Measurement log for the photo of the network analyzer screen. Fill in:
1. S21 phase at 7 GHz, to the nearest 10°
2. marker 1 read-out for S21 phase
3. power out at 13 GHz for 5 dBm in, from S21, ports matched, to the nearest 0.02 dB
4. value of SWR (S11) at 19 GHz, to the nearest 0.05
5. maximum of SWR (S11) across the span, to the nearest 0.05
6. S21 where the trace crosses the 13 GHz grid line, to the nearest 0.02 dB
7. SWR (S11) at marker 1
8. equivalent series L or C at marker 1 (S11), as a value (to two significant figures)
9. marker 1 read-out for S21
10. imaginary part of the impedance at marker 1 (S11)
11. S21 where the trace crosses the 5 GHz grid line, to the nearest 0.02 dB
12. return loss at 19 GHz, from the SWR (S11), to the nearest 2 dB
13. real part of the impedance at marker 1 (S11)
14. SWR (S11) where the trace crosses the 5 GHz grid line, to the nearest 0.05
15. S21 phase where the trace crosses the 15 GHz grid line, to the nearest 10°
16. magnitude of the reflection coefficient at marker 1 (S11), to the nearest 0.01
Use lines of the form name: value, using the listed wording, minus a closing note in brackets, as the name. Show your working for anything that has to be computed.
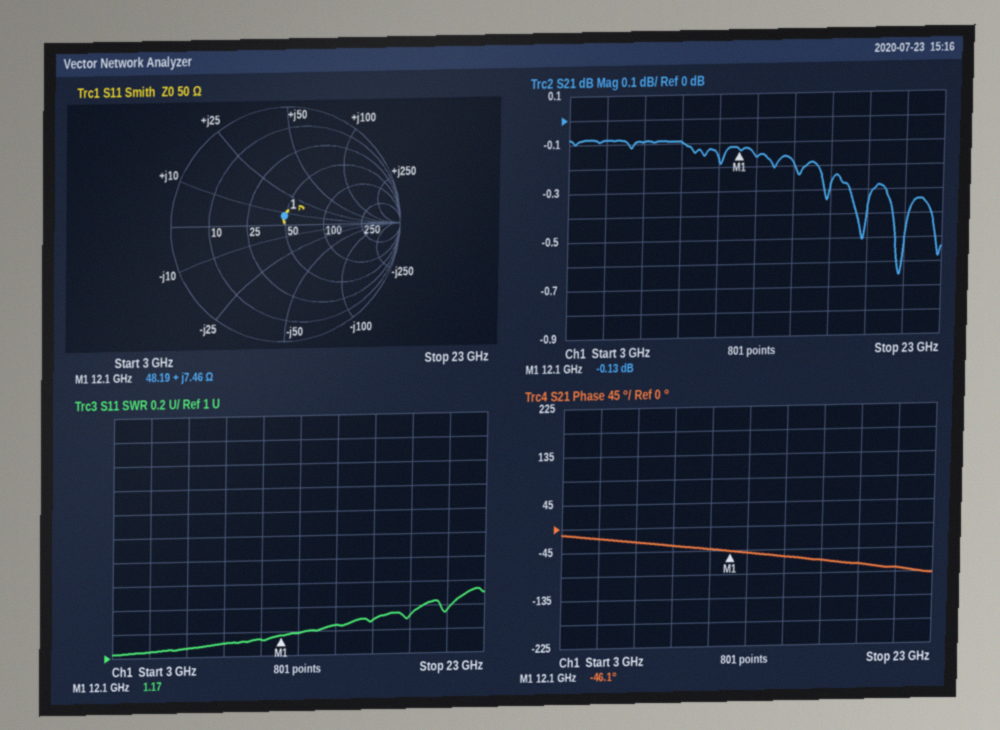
S21 phase at 7 GHz, to the nearest 10°: -30°
marker 1 read-out for S21 phase: -46.1°
power out at 13 GHz for 5 dBm in, from S21, ports matched, to the nearest 0.02 dB: 5 dBm + (-0.16 dB) = 4.84 dBm
value of SWR (S11) at 19 GHz, to the nearest 0.05: 1.30
maximum of SWR (S11) across the span, to the nearest 0.05: 1.55
S21 where the trace crosses the 13 GHz grid line, to the nearest 0.02 dB: -0.16 dB
SWR (S11) at marker 1: 1.17
equivalent series L or C at marker 1 (S11), as a value: L = 7.46 Ω/(2π × 12.1 GHz) ≈ 98 pH
marker 1 read-out for S21: -0.13 dB
imaginary part of the impedance at marker 1: +7.46 Ω
S21 where the trace crosses the 5 GHz grid line, to the nearest 0.02 dB: -0.08 dB
return loss at 19 GHz, from the SWR (S11), to the nearest 2 dB: −20 log10((1.3 − 1)/(1.3 + 1)) ≈ 18 dB
real part of the impedance at marker 1: 48.19 Ω
SWR (S11) where the trace crosses the 5 GHz grid line, to the nearest 0.05: 1.05
S21 phase where the trace crosses the 15 GHz grid line, to the nearest 10°: -60°
magnitude of the reflection coefficient at marker 1 (S11), to the nearest 0.01: 0.08
